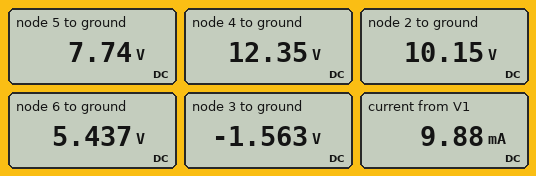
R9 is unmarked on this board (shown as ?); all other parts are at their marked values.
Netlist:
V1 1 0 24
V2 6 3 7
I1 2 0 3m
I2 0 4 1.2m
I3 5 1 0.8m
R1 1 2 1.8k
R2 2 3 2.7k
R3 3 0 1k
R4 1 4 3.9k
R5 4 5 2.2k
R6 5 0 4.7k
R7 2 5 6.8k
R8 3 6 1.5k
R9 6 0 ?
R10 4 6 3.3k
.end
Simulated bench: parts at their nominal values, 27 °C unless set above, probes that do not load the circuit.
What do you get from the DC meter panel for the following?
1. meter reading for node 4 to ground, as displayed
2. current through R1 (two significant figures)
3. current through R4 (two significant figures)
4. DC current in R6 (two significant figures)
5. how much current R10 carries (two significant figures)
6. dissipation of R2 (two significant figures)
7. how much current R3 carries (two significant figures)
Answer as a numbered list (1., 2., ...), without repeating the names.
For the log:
1. 12.35 V
2. 7.7 mA
3. 3.0 mA
4. 1.6 mA
5. 2.1 mA
6. 51 mW
7. 1.6 mA
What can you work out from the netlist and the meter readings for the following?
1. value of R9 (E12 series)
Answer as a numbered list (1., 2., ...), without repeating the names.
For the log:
1. 680 Ω
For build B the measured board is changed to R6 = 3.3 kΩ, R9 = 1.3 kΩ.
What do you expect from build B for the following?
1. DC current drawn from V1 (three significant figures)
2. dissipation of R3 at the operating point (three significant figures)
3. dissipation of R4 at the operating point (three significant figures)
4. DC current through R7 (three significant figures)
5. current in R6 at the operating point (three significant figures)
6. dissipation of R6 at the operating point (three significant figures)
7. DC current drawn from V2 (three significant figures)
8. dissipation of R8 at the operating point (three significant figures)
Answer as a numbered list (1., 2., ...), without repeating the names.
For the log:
1. 9.54 mA
2. 10.8 µW
3. 33.4 mW
4. 511 µA
5. 2.17 mA
6. 15.6 mW
7. 8.47 mA
8. 32.7 mW
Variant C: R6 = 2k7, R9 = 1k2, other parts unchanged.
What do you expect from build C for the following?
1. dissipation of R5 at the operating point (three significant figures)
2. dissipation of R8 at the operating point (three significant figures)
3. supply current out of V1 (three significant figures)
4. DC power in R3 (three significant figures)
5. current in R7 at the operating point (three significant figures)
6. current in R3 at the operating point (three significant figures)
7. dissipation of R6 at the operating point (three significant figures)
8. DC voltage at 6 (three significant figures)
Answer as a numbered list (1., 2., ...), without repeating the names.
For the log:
1. 14.9 mW
2. 32.7 mW
3. 9.75 mA
4. 23.4 µW
5. 588 µA
6. 153 µA
7. 15.5 mW
8. 6.85 V
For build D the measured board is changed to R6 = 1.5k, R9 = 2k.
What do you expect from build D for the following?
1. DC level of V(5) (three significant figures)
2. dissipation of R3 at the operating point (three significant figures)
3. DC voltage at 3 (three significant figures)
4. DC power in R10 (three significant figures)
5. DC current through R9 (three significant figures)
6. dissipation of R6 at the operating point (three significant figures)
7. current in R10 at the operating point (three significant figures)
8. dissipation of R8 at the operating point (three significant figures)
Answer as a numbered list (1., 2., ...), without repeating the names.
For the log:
1. 4.81 V
2. 734 µW
3. 857 mV
4. 4.61 mW
5. 3.93 mA
6. 15.4 mW
7. 1.18 mA
8. 32.7 mW
